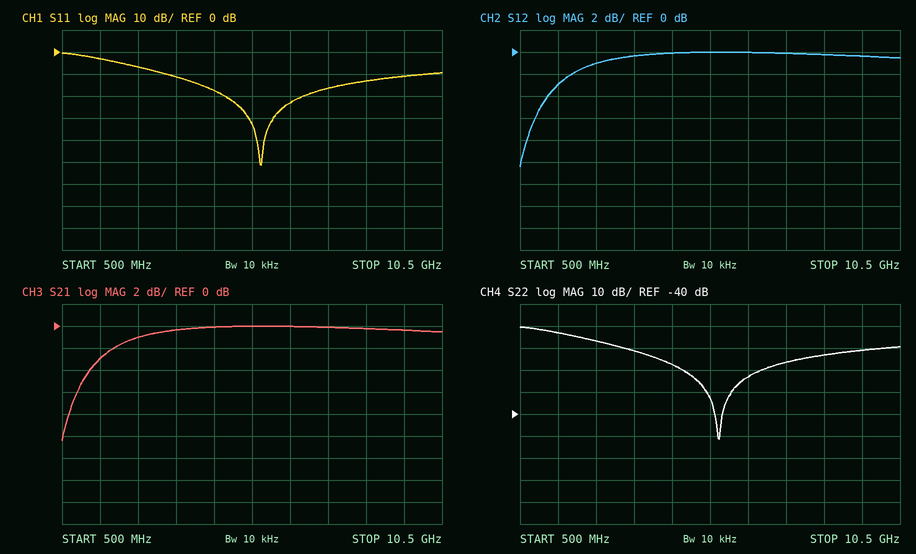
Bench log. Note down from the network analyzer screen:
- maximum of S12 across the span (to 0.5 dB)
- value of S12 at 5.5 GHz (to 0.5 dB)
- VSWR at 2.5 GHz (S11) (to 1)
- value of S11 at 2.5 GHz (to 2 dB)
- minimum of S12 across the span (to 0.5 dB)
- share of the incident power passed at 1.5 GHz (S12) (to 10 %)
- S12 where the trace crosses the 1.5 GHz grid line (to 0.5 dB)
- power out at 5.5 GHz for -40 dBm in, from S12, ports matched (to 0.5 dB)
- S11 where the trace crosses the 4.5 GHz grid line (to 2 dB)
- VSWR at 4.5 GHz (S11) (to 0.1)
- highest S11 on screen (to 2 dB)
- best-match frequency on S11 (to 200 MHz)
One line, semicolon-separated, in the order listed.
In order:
0.0 dB; 0.0 dB; 3; -6 dB; -10.5 dB; 50 %; -3.0 dB; -40.0 dBm; -18 dB; 1.3; 0 dB; 5.8 GHz
